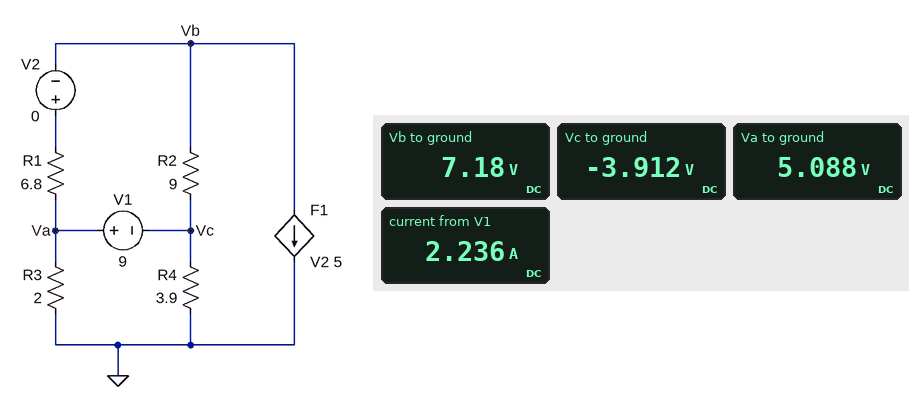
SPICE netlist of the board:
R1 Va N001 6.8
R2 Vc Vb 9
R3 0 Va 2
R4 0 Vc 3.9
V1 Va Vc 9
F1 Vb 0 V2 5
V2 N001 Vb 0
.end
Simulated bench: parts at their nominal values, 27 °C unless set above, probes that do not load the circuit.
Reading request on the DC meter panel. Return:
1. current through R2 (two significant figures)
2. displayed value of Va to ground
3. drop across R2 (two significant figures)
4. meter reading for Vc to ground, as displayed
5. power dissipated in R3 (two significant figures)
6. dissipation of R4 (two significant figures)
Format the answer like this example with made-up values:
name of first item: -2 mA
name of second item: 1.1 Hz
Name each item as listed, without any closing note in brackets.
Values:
current through R2: 1.2 A
displayed value of Va to ground: 5.088 V
drop across R2: 11 V
meter reading for Vc to ground, as displayed: -3.912 V
power dissipated in R3: 13 W
dissipation of R4: 3.9 W
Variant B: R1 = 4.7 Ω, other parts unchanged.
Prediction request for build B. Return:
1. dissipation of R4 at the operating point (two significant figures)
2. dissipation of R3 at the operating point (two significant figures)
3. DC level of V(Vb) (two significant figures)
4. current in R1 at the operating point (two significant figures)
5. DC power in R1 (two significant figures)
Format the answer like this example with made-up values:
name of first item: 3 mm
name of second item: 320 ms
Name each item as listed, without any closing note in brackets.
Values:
dissipation of R4 at the operating point: 4.2 W
dissipation of R3 at the operating point: 12 W
DC level of V(Vb): 6.3 V
current in R1 at the operating point: 290 mA
DC power in R1: 390 mW
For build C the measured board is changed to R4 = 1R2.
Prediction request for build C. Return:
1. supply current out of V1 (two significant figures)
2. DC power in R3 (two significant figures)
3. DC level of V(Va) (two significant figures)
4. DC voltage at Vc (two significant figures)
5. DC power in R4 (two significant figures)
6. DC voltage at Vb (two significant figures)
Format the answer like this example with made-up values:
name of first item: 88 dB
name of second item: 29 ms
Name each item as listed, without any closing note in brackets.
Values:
supply current out of V1: 3.1 A
DC power in R3: 23 W
DC level of V(Va): 6.8 V
DC voltage at Vc: -2.2 V
DC power in R4: 4.1 W
DC voltage at Vb: 8.9 V
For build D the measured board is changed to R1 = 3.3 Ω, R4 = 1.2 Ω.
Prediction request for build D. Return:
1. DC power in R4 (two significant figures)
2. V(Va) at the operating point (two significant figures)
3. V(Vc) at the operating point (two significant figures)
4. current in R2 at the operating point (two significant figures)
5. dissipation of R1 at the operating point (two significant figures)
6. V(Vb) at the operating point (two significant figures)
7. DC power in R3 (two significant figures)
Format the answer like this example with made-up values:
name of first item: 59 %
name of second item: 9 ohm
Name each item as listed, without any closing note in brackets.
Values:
DC power in R4: 4.6 W
V(Va) at the operating point: 6.7 V
V(Vc) at the operating point: -2.3 V
current in R2 at the operating point: 1.1 A
dissipation of R1 at the operating point: 250 mW
V(Vb) at the operating point: 7.6 V
DC power in R3: 22 W
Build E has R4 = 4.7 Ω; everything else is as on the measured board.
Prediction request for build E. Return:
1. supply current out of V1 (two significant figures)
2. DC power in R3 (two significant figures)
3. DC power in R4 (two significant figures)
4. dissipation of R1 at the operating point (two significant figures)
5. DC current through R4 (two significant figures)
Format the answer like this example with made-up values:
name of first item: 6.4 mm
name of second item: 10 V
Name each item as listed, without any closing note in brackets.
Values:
supply current out of V1: 2.1 A
DC power in R3: 12 W
DC power in R4: 3.7 W
dissipation of R1 at the operating point: 650 mW
DC current through R4: 880 mA
